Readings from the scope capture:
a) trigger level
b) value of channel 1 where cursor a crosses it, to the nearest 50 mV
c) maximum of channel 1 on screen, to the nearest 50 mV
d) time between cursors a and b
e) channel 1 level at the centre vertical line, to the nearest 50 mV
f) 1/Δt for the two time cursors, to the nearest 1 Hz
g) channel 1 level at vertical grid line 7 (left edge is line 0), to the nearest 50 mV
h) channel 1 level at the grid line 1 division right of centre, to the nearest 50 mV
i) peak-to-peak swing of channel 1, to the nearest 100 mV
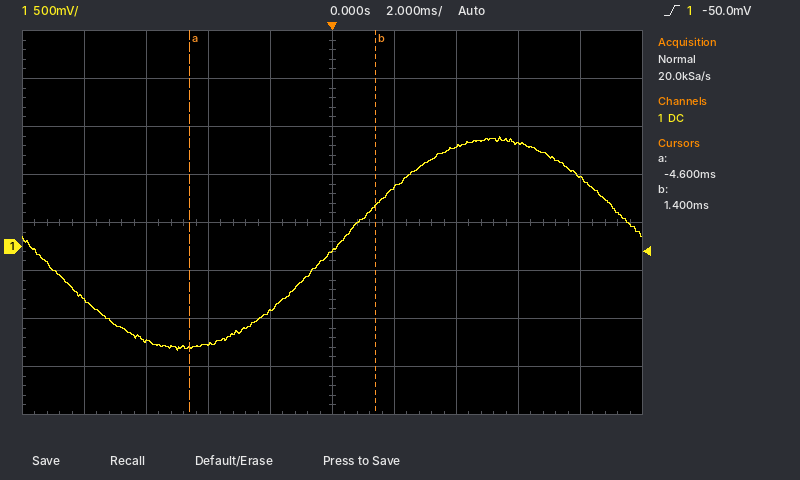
-50.0 mV
-1.05 V
1.15 V
6.0 ms
-50 mV
167 Hz
1.05 V
600 mV
2.20 V
